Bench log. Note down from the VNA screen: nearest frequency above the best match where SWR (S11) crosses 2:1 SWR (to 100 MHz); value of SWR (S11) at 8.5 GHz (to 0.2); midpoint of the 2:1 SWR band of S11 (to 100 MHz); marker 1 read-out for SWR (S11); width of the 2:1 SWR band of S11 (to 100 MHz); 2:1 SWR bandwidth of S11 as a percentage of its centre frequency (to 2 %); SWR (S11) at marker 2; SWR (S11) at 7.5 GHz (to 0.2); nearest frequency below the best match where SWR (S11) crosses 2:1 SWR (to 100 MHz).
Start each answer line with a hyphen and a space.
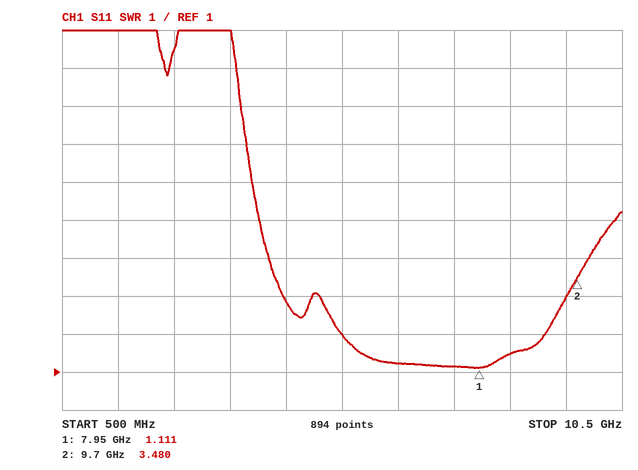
- 9.1 GHz
- 1.4
- 7.3 GHz
- 1.111
- 3.6 GHz
- 50 %
- 3.480
- 1.2
- 5.5 GHz
